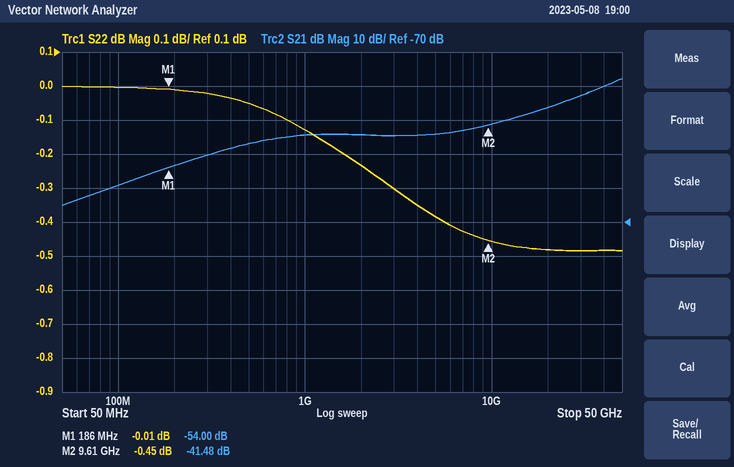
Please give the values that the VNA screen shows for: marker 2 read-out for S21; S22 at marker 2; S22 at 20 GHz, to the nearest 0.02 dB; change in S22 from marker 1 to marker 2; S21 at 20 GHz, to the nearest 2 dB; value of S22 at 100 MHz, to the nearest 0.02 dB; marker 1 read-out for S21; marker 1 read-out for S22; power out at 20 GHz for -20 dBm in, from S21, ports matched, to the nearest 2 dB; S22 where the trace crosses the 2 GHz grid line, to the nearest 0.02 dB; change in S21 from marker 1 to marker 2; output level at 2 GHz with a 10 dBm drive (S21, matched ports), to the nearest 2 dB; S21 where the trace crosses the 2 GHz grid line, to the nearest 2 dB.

-41.48 dB
-0.45 dB
-0.48 dB
-0.44 dB
-36 dB
0.00 dB
-54.00 dB
-0.01 dB
-56 dBm
-0.24 dB
12.52 dB
-34 dBm
-44 dB
